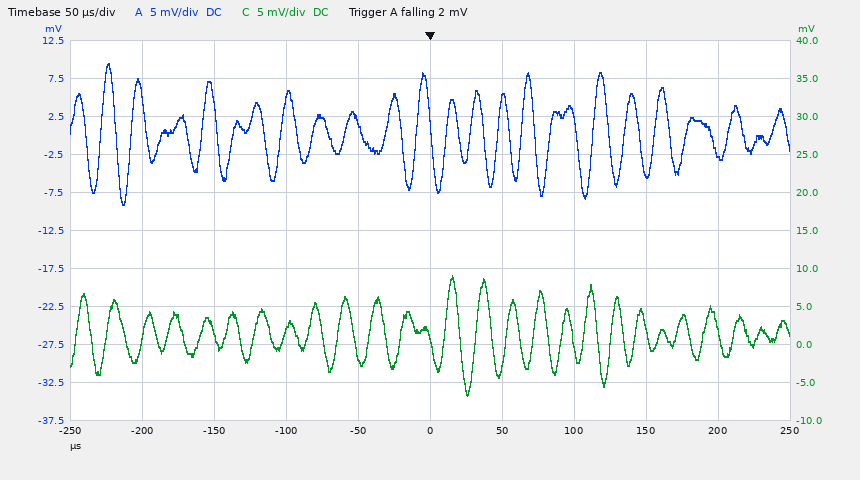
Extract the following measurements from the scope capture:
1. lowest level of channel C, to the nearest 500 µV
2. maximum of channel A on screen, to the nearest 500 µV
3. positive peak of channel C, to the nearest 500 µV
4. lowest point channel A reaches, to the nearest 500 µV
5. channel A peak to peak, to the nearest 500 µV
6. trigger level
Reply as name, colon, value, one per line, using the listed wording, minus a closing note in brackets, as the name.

lowest level of channel C, to the nearest 500 µV: -6.5 mV
maximum of channel A on screen, to the nearest 500 µV: 9.5 mV
positive peak of channel C, to the nearest 500 µV: 9.0 mV
lowest point channel A reaches, to the nearest 500 µV: -9.0 mV
channel A peak to peak, to the nearest 500 µV: 18.5 mV
trigger level: 2 mV
